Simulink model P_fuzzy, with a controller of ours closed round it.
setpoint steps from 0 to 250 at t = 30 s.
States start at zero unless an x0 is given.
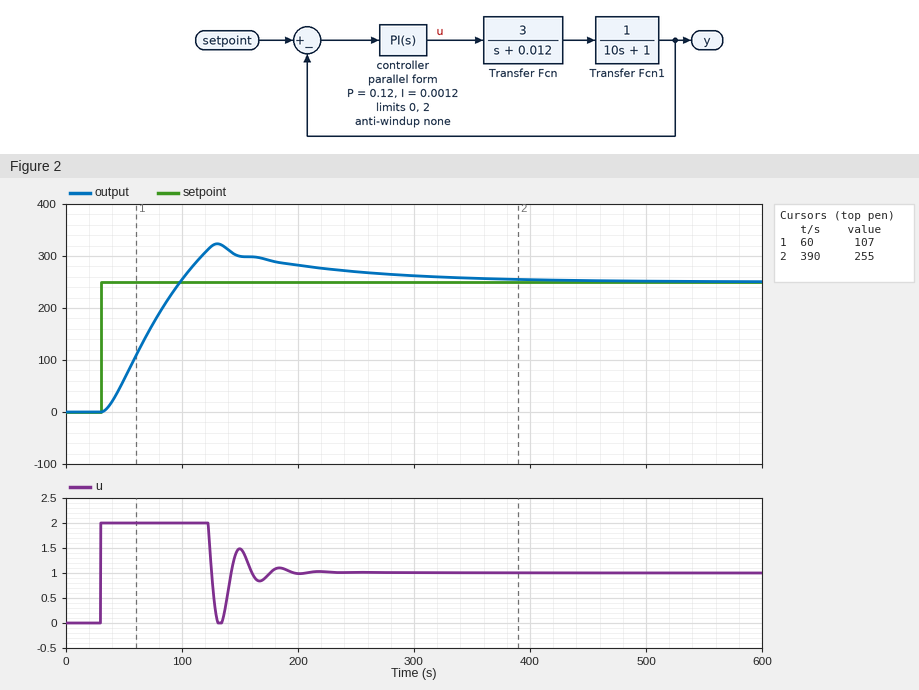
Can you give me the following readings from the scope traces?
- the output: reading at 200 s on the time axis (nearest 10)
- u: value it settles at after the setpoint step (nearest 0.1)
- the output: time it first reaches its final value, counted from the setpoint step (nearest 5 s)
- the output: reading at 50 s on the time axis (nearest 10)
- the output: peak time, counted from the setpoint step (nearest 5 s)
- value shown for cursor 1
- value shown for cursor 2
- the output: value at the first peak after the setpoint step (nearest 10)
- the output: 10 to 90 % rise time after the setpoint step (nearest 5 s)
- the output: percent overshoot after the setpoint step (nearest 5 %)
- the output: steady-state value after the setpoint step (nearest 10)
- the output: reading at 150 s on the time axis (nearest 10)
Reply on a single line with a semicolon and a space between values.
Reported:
280; 1.0; 70 s; 60; 100 s; 107; 255; 320; 50 s; 30 %; 250; 300
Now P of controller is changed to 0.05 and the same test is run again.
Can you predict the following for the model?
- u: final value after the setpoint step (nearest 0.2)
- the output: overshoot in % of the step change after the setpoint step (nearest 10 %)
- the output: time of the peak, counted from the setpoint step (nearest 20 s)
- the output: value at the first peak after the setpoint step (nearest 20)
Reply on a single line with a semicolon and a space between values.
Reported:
1.0; 50 %; 120 s; 360
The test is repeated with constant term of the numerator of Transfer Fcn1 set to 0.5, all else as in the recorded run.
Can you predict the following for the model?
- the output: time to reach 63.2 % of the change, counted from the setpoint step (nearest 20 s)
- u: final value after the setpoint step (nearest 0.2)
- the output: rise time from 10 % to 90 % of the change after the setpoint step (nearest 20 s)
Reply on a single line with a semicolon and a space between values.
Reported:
100 s; 2.0; 180 s
